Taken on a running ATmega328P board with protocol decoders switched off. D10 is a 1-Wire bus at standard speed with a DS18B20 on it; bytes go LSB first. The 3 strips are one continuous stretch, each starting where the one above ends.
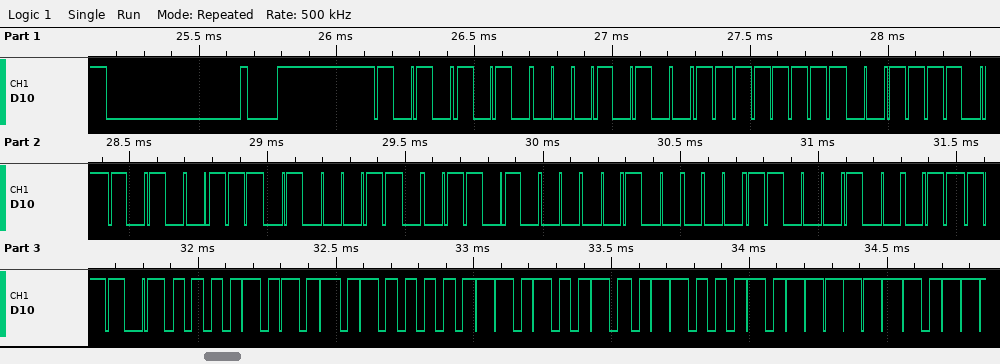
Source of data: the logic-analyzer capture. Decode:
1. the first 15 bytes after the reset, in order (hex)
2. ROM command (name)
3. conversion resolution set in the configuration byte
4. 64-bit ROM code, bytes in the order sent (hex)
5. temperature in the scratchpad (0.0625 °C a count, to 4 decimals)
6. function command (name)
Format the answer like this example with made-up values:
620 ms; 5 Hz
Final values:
55 28 FF BC E5 62 16 04 23 BE 50 05 4B 46 7F; Match ROM; 12 bits; 28 FF BC E5 62 16 04 23; 85.0000 °C; Read Scratchpad
